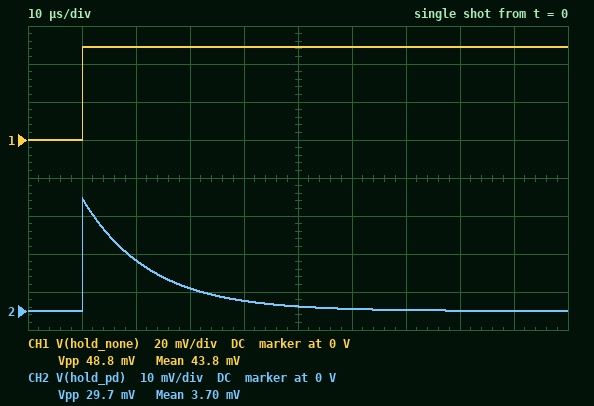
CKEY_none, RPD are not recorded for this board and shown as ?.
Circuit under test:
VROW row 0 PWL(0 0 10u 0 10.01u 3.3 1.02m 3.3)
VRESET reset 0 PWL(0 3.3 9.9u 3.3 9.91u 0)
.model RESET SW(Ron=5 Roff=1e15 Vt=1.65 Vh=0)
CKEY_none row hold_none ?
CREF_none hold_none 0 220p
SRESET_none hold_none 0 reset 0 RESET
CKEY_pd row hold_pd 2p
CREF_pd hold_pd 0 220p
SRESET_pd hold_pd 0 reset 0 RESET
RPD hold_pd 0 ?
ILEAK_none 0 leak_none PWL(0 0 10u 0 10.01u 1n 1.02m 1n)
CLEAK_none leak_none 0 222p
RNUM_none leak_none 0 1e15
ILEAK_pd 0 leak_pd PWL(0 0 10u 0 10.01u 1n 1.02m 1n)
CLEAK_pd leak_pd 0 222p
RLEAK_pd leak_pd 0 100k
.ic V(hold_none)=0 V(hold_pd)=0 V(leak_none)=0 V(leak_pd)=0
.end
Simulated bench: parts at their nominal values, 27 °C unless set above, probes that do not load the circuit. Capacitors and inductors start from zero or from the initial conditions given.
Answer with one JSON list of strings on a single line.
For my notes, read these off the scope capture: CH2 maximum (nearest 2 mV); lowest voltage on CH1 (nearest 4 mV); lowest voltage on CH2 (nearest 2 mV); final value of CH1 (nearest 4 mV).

["30 mV", "0 V", "0 V", "48 mV"]
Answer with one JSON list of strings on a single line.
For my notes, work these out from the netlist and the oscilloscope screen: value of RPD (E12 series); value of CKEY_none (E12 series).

["56 kΩ", "3.3 pF"]
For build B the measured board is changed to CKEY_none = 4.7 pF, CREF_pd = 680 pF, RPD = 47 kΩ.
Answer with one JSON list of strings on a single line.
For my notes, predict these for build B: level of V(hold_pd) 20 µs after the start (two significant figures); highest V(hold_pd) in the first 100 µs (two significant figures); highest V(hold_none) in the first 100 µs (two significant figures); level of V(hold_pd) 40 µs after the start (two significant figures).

["7.1 mV", "9.7 mV", "69 mV", "3.8 mV"]
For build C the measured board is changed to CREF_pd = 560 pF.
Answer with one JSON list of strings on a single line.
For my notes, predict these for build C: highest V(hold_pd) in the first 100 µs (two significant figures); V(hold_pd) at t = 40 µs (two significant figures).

["12 mV", "4.5 mV"]
